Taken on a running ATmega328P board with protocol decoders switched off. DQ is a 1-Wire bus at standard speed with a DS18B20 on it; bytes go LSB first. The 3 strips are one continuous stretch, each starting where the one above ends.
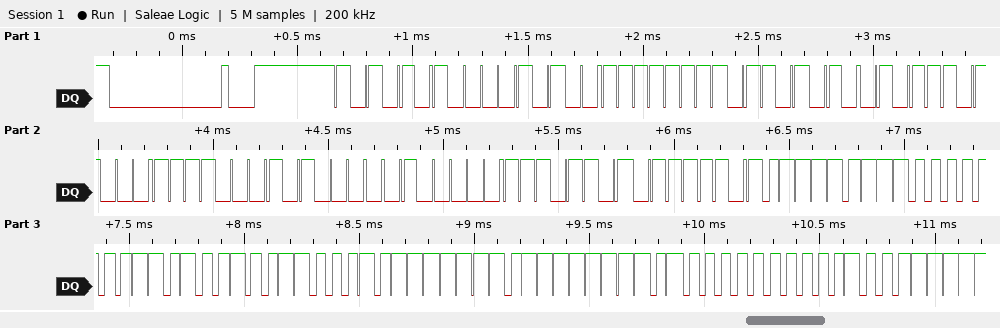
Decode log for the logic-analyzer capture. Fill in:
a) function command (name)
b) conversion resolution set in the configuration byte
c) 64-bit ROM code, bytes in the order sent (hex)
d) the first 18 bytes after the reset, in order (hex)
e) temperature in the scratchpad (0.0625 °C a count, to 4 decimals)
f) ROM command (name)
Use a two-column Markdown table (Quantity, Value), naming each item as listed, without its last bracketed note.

| Quantity | Value |
|---|---|
| function command | Read Scratchpad |
| conversion resolution set in the configuration byte | 12 bits |
| 64-bit ROM code, bytes in the order sent | 28 FF 56 BA 78 14 04 B7 |
| the first 18 bytes after the reset, in order | 55 28 FF 56 BA 78 14 04 B7 BE DE 01 4B 46 7F FF 02 10 |
| temperature in the scratchpad | 29.8750 °C |
| ROM command | Match ROM |
